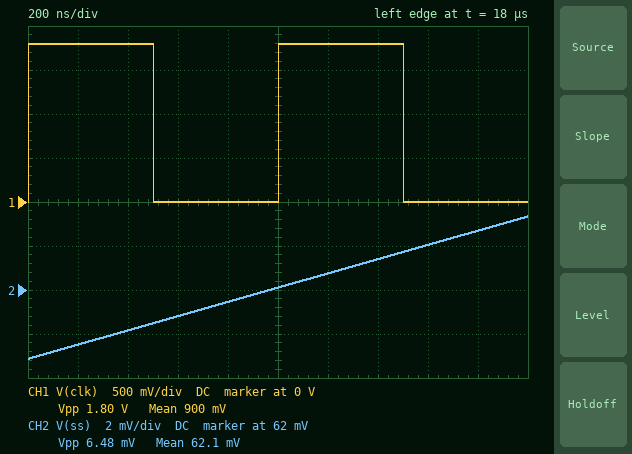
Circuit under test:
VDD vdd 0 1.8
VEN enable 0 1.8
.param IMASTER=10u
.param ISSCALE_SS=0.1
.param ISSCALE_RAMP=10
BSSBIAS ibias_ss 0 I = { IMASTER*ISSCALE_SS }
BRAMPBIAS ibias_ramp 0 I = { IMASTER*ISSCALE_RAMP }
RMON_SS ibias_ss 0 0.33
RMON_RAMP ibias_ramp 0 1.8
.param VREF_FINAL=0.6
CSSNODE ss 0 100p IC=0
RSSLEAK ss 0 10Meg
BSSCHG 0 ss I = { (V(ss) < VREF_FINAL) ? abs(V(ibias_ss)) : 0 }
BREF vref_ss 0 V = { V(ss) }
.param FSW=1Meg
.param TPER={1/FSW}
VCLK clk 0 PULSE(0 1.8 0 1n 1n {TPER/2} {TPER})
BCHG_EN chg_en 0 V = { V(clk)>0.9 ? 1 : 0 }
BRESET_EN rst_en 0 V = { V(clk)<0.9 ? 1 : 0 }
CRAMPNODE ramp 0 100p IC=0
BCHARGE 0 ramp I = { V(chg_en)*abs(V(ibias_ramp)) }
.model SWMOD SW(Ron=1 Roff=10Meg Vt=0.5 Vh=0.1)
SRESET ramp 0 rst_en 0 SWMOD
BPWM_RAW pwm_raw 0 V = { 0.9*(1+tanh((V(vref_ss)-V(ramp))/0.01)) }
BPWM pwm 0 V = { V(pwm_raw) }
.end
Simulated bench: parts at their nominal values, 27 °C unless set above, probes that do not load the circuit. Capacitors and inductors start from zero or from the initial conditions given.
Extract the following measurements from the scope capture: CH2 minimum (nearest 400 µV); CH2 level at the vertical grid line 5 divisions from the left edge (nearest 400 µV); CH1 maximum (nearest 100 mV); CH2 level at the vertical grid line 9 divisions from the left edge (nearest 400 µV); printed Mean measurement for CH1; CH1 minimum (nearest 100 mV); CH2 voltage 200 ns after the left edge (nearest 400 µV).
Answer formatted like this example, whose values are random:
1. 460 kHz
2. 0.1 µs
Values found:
1. 58.8 mV
2. 62.0 mV
3. 1.8 V
4. 64.8 mV
5. 900 mV
6. 0 V
7. 59.6 mV
